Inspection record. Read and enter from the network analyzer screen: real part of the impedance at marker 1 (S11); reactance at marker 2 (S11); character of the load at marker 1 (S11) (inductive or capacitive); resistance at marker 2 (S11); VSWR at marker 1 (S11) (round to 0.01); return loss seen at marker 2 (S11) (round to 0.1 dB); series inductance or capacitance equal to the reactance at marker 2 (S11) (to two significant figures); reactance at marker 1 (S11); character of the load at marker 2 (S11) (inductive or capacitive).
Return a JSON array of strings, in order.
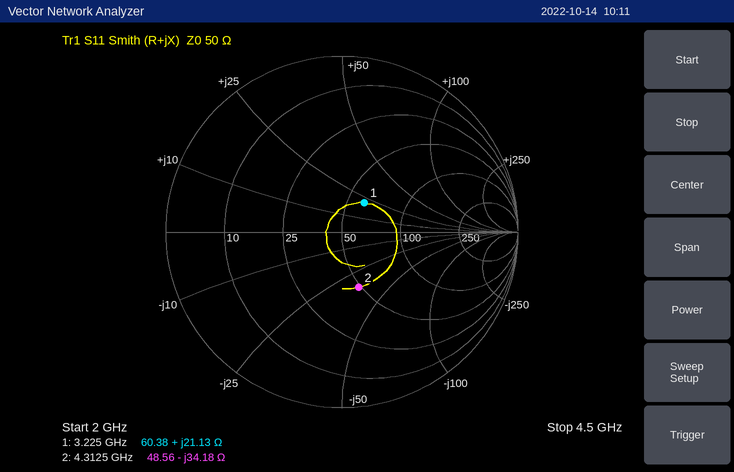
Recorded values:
["60.38 Ω", "-34.18 Ω", "inductive", "48.56 Ω", "1.53", "9.7 dB", "1.1 pF", "+21.13 Ω", "capacitive"]
